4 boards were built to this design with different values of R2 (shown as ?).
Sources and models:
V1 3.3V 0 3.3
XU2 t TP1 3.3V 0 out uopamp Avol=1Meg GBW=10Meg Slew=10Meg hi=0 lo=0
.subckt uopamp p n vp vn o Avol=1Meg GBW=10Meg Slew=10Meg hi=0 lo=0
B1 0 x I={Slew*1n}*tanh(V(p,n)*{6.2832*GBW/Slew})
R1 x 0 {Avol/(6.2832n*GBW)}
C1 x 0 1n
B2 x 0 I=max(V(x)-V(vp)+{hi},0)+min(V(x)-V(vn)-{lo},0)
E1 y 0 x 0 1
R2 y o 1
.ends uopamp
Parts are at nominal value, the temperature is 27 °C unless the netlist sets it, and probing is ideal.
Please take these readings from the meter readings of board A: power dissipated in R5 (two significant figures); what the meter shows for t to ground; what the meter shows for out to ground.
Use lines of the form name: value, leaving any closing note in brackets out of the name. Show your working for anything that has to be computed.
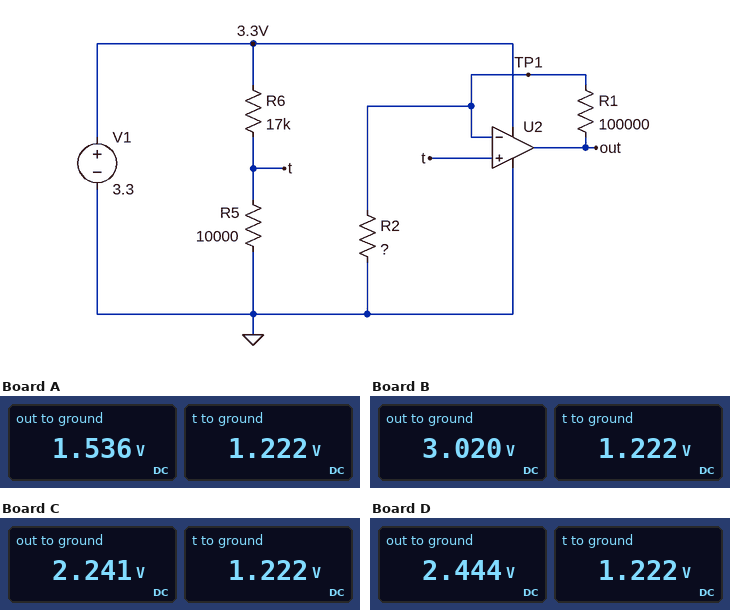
power dissipated in R5: (1.222 V)^2 / 10 kΩ = 150 µW
what the meter shows for t to ground: 1.222 V
what the meter shows for out to ground: 1.536 V
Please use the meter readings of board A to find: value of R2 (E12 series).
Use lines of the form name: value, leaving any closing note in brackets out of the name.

value of R2: 390 kΩ
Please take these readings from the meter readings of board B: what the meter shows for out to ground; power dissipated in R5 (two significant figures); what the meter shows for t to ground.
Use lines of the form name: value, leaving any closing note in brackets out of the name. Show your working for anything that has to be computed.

what the meter shows for out to ground: 3.020 V
power dissipated in R5: (1.222 V)^2 / 10 kΩ = 150 µW
what the meter shows for t to ground: 1.222 V
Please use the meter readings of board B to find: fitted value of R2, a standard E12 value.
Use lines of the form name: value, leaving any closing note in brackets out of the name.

fitted value of R2, a standard E12 value: 68 kΩ
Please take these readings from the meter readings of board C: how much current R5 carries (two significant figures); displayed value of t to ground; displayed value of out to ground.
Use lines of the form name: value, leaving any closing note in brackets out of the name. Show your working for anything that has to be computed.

how much current R5 carries: (1.222 V) / 10 kΩ = 120 µA
displayed value of t to ground: 1.222 V
displayed value of out to ground: 2.241 V
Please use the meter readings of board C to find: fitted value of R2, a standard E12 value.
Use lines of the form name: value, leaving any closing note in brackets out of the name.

fitted value of R2, a standard E12 value: 120 kΩ
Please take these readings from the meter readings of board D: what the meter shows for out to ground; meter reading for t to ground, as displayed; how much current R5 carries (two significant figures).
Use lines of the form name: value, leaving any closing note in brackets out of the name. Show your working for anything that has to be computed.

what the meter shows for out to ground: 2.444 V
meter reading for t to ground, as displayed: 1.222 V
how much current R5 carries: (1.222 V) / 10 kΩ = 120 µA
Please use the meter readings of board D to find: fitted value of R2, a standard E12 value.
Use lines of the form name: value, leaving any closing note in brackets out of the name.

fitted value of R2, a standard E12 value: 100 kΩ
